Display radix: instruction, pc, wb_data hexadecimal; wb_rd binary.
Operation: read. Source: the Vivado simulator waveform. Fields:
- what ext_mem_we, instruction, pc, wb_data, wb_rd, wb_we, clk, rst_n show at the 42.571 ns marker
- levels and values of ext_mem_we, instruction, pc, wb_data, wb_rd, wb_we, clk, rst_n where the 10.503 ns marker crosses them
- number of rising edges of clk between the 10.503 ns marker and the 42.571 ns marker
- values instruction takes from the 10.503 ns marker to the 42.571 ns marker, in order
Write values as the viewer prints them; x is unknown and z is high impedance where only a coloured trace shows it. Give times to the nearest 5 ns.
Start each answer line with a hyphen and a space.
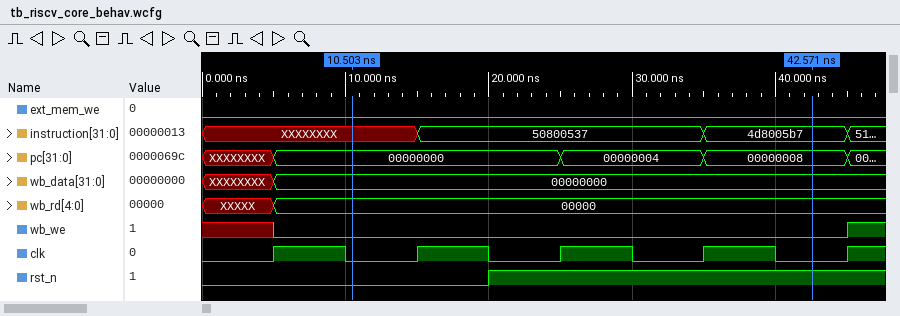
- ext_mem_we=0, instruction=4d8005b7, pc=00000008, wb_data=00000000, wb_rd=00000, wb_we=0, clk=0, rst_n=1
- ext_mem_we=0, instruction=XXXXXXXX, pc=00000000, wb_data=00000000, wb_rd=00000, wb_we=0, clk=0, rst_n=0
- 3
- XXXXXXXX, 50800537, 4d8005b7
